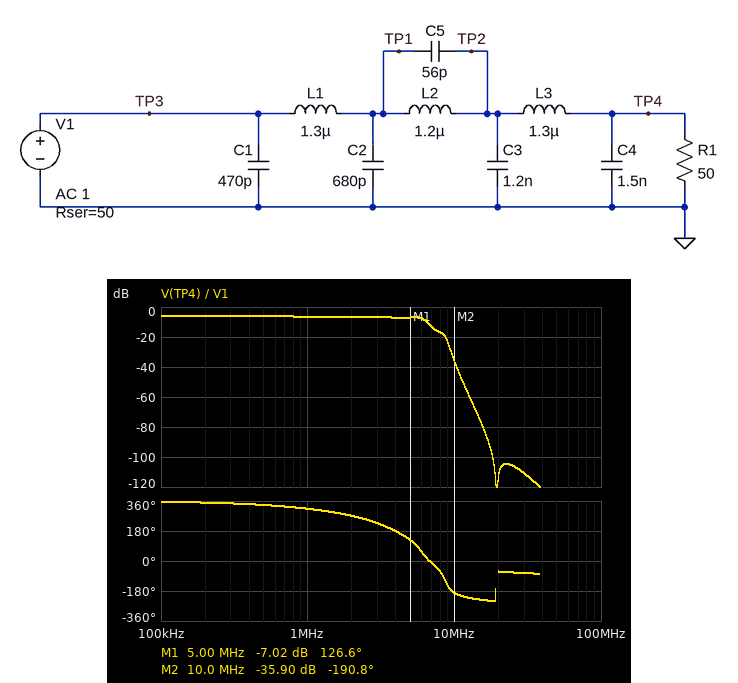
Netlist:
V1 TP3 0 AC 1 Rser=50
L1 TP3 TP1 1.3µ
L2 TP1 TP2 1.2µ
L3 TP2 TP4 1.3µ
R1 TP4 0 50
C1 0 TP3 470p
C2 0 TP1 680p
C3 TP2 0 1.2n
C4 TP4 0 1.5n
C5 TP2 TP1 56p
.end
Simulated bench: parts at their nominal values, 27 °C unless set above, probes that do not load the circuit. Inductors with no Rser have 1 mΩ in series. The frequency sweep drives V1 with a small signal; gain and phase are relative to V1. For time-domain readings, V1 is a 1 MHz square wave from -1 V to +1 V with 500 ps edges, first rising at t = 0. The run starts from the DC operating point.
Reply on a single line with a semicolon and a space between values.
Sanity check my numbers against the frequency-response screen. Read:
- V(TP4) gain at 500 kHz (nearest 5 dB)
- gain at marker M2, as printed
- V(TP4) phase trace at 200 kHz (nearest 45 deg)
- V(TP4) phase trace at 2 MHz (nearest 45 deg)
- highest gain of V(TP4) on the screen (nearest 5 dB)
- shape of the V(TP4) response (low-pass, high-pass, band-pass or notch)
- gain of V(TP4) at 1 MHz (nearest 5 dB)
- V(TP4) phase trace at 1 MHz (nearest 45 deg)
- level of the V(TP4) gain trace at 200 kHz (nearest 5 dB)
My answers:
-5 dB; -35.90 dB; 360 deg; 270 deg; -5 dB; low-pass; -5 dB; 315 deg; -5 dB
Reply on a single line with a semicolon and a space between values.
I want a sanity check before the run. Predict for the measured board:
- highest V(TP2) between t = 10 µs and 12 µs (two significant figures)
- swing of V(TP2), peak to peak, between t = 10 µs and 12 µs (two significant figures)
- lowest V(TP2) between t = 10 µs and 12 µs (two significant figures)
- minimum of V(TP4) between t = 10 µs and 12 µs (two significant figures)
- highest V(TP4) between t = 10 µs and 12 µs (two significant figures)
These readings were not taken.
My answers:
620 mV; 1.2 V; -620 mV; -580 mV; 580 mV
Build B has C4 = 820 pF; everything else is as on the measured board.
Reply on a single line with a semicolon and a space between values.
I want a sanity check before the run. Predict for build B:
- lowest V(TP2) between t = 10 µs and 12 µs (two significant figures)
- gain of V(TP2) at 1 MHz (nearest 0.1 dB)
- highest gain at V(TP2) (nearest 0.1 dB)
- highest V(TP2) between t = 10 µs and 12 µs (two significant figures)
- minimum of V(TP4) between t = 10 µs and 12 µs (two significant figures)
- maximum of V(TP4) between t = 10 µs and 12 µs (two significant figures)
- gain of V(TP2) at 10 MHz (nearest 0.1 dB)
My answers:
-600 mV; -6.5 dB; -4.4 dB; 600 mV; -640 mV; 640 mV; -18.9 dB
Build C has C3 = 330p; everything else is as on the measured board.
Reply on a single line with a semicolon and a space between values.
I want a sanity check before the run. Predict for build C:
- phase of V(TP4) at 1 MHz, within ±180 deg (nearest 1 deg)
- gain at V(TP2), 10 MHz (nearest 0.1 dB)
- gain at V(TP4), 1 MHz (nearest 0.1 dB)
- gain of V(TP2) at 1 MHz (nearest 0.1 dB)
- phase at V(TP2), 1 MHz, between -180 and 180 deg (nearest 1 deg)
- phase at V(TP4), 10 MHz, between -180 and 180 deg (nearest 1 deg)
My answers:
-40 deg; -4.3 dB; -6.2 dB; -6.8 dB; -30 deg; -25 deg
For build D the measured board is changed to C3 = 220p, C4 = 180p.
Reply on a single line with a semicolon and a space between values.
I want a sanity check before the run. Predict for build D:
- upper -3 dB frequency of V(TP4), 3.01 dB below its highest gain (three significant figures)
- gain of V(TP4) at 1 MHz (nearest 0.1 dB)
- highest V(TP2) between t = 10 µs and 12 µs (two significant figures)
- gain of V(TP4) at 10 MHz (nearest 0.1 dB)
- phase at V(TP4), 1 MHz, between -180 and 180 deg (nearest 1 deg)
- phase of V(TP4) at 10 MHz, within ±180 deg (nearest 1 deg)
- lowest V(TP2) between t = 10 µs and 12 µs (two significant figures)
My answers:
8.59 MHz; -6.0 dB; 690 mV; -14.0 dB; -28 deg; 32 deg; -690 mV
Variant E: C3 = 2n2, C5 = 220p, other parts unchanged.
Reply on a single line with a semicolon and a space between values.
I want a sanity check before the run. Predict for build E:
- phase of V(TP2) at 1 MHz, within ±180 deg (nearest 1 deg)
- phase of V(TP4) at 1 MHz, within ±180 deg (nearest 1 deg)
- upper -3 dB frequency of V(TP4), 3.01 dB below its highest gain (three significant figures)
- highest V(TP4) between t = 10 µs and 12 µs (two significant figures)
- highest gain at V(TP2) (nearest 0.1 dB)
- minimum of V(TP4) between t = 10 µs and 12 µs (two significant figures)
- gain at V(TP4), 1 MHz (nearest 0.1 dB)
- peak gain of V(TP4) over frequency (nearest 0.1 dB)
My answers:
-44 deg; -54 deg; 5.22 MHz; 560 mV; -5.5 dB; -560 mV; -6.9 dB; -6.0 dB
